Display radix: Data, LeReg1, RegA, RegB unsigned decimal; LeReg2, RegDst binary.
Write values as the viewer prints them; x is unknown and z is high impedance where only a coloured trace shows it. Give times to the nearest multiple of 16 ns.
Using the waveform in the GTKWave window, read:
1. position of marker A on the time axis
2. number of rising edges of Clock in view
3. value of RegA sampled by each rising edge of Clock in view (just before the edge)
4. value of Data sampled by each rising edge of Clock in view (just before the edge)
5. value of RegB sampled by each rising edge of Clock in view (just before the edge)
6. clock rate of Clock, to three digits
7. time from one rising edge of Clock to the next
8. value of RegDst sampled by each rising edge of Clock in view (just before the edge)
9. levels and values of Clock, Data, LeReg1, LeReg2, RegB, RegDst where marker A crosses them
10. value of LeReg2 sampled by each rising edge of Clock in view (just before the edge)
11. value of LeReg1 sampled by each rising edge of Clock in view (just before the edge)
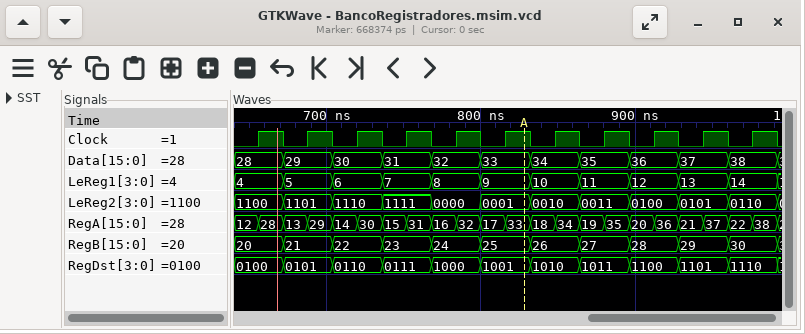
832 ns
11
12, 13, 14, 15, 16, 17, 18, 19, 20, 21, 22
28, 29, 30, 31, 32, 33, 34, 35, 36, 37, 38
20, 21, 22, 23, 24, 25, 26, 27, 28, 29, 30
31.2 MHz
32 ns
0100, 0101, 0110, 0111, 1000, 1001, 1010, 1011, 1100, 1101, 1110
Clock=1, Data=33, LeReg1=9, LeReg2=0001, RegB=25, RegDst=1001
1100, 1101, 1110, 1111, 0000, 0001, 0010, 0011, 0100, 0101, 0110
4, 5, 6, 7, 8, 9, 10, 11, 12, 13, 14
